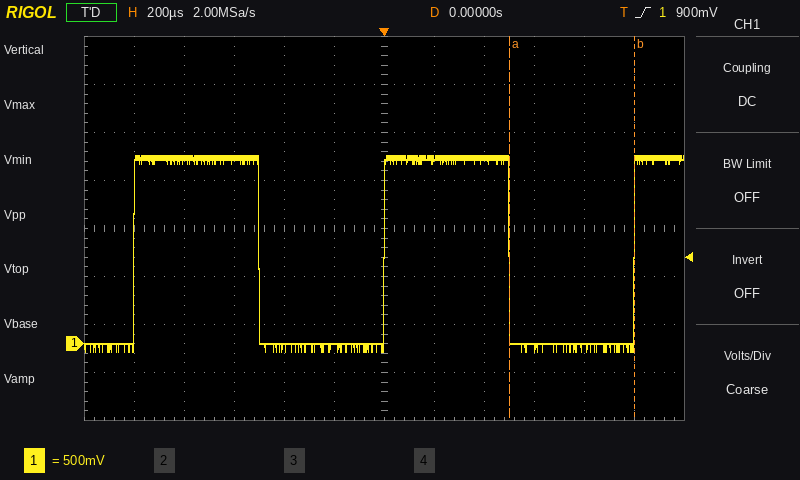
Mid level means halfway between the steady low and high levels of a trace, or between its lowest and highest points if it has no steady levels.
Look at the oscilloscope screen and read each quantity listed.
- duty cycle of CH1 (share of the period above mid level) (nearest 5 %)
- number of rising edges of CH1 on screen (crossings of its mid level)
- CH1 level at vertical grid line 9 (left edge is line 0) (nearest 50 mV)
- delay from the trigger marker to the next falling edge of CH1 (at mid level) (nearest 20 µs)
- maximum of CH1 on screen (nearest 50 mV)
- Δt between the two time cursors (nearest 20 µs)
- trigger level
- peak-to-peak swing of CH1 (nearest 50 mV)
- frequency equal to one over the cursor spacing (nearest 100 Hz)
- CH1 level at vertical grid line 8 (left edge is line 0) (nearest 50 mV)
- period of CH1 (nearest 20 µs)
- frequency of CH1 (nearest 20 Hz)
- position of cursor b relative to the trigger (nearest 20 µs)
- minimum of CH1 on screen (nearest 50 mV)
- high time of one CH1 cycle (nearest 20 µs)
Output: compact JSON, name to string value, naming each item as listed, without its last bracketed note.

{"duty cycle of CH1 (share of the period above mid level)": "50 %", "number of rising edges of CH1 on screen": "3", "CH1 level at vertical grid line 9 (left edge is line 0)": "-50 mV", "delay from the trigger marker to the next falling edge of CH1 (at mid level)": "500 µs", "maximum of CH1 on screen": "1.95 V", "Δt between the two time cursors": "500 µs", "trigger level": "900 mV", "peak-to-peak swing of CH1": "2.05 V", "frequency equal to one over the cursor spacing": "2.0 kHz", "CH1 level at vertical grid line 8 (left edge is line 0)": "1.95 V", "period of CH1": "1.00 ms", "frequency of CH1": "1.00 kHz", "position of cursor b relative to the trigger": "+1.00 ms", "minimum of CH1 on screen": "-100 mV", "high time of one CH1 cycle": "500 µs"}
